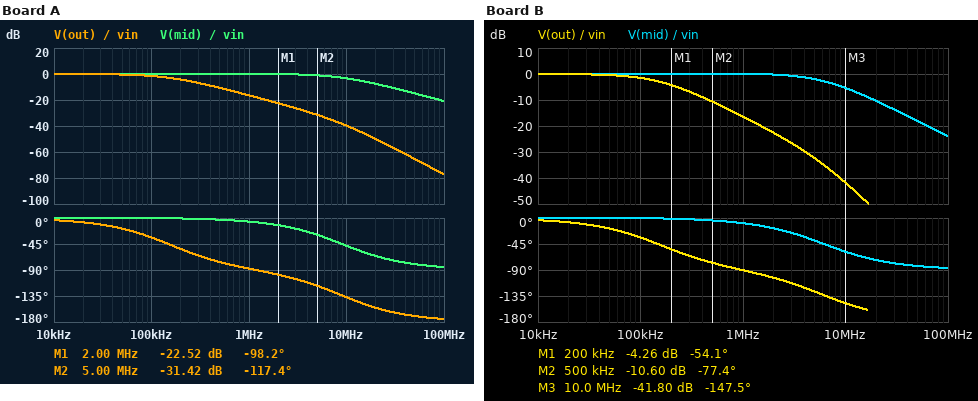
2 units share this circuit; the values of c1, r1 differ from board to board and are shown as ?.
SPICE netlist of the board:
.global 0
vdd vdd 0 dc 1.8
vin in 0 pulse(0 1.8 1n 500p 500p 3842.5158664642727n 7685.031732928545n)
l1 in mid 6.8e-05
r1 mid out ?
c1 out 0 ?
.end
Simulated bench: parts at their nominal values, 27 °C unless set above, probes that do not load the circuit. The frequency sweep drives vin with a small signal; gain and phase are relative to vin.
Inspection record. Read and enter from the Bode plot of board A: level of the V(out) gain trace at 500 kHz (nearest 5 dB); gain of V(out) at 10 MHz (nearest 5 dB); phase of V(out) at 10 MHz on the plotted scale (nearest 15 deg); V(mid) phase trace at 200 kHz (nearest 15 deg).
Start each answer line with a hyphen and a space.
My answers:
- -10 dB
- -40 dB
- -135 deg
- 0 deg
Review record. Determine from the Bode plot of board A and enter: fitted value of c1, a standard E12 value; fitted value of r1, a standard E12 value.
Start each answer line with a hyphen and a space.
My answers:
- 270 pF
- 3.9 kΩ
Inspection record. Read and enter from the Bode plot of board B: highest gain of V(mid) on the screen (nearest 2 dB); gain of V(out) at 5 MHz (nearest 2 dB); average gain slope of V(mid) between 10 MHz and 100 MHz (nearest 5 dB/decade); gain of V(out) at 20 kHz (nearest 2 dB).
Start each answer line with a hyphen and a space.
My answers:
- 0 dB
- -32 dB
- -20 dB/decade
- 0 dB
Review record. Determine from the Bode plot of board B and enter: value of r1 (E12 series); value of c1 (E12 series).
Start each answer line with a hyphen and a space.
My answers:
- 2.7 kΩ
- 390 pF
